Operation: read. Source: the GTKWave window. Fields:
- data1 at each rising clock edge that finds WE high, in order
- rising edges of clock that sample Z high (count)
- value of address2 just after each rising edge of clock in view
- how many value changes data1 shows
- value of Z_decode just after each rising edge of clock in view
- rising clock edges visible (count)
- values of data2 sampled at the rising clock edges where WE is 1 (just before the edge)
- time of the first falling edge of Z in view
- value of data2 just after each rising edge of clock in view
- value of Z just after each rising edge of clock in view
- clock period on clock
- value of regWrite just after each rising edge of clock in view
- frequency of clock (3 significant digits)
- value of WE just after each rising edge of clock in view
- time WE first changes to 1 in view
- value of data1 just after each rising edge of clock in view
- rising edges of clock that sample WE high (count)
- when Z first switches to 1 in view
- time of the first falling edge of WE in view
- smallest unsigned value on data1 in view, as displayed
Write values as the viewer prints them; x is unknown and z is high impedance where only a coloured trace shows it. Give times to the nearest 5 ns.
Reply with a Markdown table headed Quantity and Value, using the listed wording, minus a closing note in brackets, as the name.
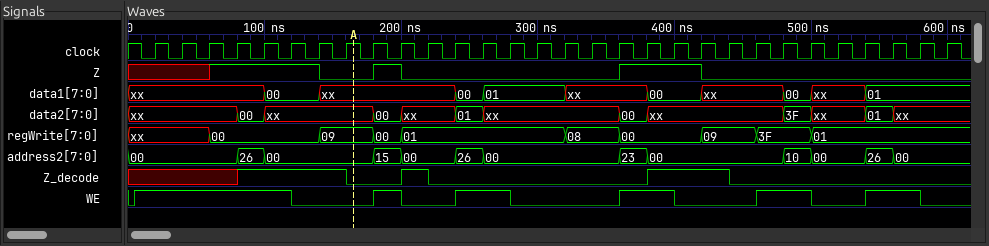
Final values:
| Quantity | Value |
|---|---|
| data1 at each rising clock edge that finds WE high, in order | xx, xx, xx, xx, xx, 00, xx, 00, 01, xx, 00, xx, 00, 01, 01 |
| rising edges of clock that sample Z high | 8 |
| value of address2 just after each rising edge of clock in view | 00, 00, 00, 26, 00, 00, 00, 00, 15, 00, 00, 26, 00, 00, 00, 00, 00, 23, 00, 00, 00, 00, 00, 10, 00, 00, 26, 00, 00, 00 |
| how many value changes data1 shows | 10 |
| value of Z_decode just after each rising edge of clock in view | x x x 1 1 1 1 0 0 1 0 0 0 0 0 0 0 0 1 1 1 0 0 0 0 0 0 0 0 0 |
| rising clock edges visible | 30 |
| values of data2 sampled at the rising clock edges where WE is 1 | xx, xx, xx, xx, 00, xx, 00, 01, xx, 00, xx, xx, 3F, 01, xx |
| time of the first falling edge of Z in view | 140 ns |
| value of data2 just after each rising edge of clock in view | xx, xx, xx, 00, xx, xx, xx, xx, 00, xx, xx, 01, xx, xx, xx, xx, xx, 00, xx, xx, xx, xx, xx, 3F, xx, xx, 01, xx, xx, xx |
| value of Z just after each rising edge of clock in view | x x 1 1 1 1 0 0 1 0 0 0 0 0 0 0 0 1 1 1 0 0 0 0 0 0 0 0 0 0 |
| clock period on clock | 20 ns |
| value of regWrite just after each rising edge of clock in view | xx, xx, 00, 00, 00, 00, 09, 09, 00, 01, 01, 01, 01, 01, 01, 08, 08, 00, 00, 00, 09, 09, 3F, 3F, 01, 01, 01, 01, 01, 01 |
| frequency of clock | 50.0 MHz |
| value of WE just after each rising edge of clock in view | 1 1 1 1 1 0 0 0 1 0 0 1 1 0 0 0 0 1 1 0 0 0 1 1 0 0 1 1 0 0 |
| time WE first changes to 1 in view | 5 ns |
| value of data1 just after each rising edge of clock in view | xx, xx, xx, xx, 00, 00, xx, xx, xx, xx, xx, 00, 01, 01, 01, xx, xx, xx, 00, 00, xx, xx, xx, 00, xx, xx, 01, 01, 01, 01 |
| rising edges of clock that sample WE high | 15 |
| when Z first switches to 1 in view | 60 ns |
| time of the first falling edge of WE in view | 120 ns |
| smallest unsigned value on data1 in view, as displayed | 00 |
